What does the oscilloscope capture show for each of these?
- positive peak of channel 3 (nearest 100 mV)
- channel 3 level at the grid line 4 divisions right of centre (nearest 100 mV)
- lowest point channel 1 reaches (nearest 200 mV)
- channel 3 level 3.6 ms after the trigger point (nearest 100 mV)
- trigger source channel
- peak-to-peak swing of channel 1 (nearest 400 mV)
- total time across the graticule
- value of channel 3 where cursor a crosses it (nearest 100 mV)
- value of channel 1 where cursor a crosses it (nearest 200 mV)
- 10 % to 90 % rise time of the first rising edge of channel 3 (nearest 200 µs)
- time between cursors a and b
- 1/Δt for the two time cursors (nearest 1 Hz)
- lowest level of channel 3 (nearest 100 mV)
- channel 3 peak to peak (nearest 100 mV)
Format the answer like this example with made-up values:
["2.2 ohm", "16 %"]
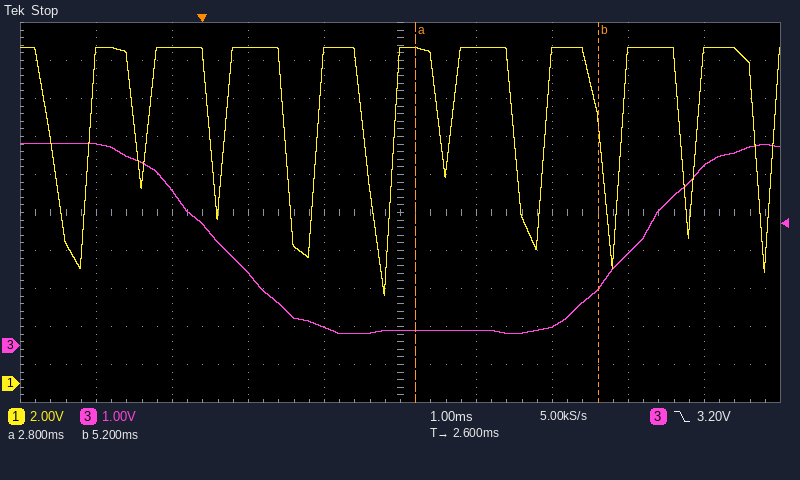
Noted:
["5.3 V", "4.7 V", "4.6 V", "400 mV", "channel 3", "13.2 V", "10 ms", "400 mV", "17.6 V", "1.8 ms", "2.4 ms", "417 Hz", "300 mV", "5.0 V"]
